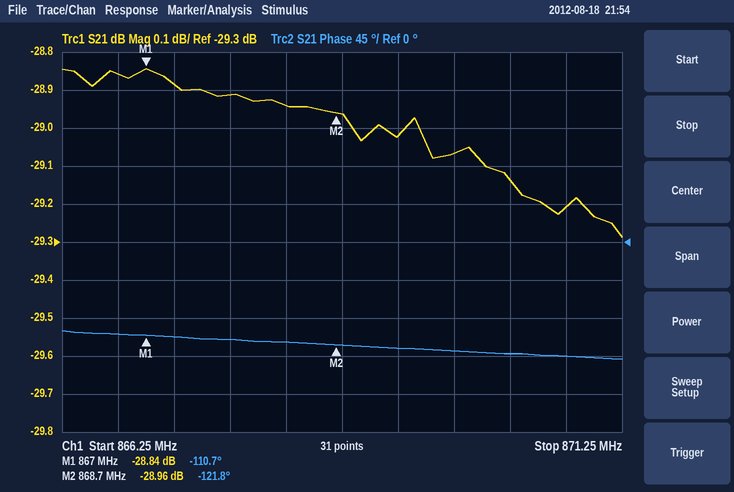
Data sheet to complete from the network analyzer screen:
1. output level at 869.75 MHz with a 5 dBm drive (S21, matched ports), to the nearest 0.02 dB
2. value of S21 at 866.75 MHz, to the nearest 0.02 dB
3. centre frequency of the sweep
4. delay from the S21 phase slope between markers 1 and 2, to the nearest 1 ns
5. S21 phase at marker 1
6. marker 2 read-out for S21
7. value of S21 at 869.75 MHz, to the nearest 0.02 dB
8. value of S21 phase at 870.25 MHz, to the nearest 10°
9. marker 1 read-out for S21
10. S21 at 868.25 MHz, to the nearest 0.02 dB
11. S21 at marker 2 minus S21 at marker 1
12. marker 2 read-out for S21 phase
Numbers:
-24.06 dBm
-28.86 dB
868.75 MHz
18 ns
-110.7°
-28.96 dB
-29.06 dB
-130°
-28.84 dB
-28.94 dB
-0.12 dB
-121.8°
